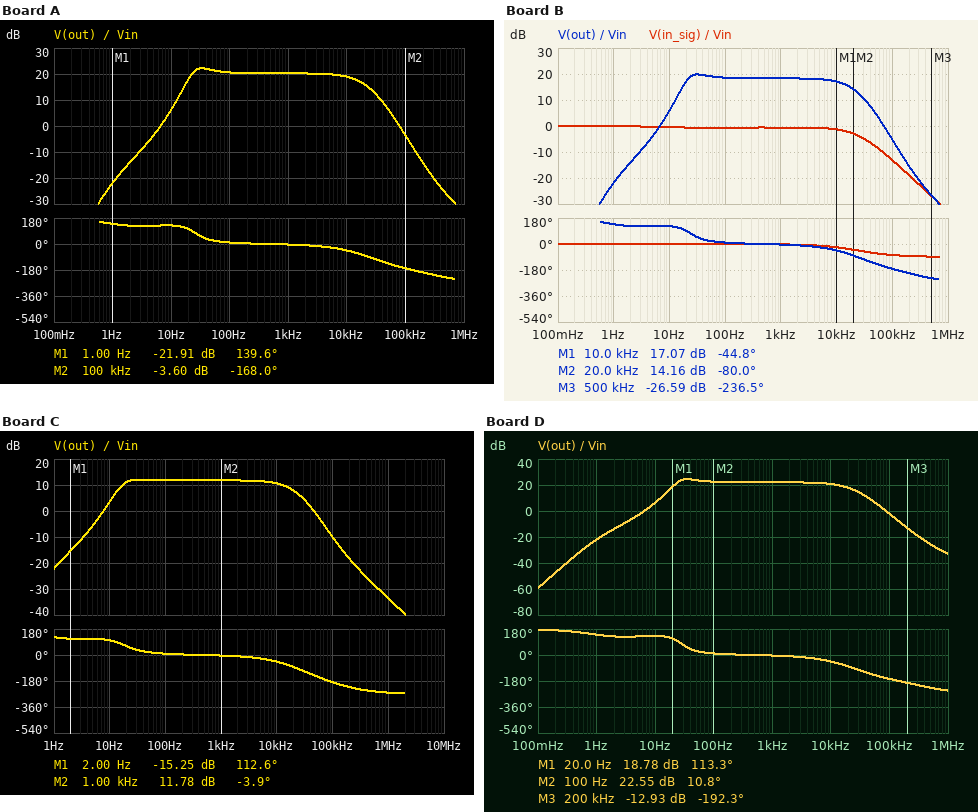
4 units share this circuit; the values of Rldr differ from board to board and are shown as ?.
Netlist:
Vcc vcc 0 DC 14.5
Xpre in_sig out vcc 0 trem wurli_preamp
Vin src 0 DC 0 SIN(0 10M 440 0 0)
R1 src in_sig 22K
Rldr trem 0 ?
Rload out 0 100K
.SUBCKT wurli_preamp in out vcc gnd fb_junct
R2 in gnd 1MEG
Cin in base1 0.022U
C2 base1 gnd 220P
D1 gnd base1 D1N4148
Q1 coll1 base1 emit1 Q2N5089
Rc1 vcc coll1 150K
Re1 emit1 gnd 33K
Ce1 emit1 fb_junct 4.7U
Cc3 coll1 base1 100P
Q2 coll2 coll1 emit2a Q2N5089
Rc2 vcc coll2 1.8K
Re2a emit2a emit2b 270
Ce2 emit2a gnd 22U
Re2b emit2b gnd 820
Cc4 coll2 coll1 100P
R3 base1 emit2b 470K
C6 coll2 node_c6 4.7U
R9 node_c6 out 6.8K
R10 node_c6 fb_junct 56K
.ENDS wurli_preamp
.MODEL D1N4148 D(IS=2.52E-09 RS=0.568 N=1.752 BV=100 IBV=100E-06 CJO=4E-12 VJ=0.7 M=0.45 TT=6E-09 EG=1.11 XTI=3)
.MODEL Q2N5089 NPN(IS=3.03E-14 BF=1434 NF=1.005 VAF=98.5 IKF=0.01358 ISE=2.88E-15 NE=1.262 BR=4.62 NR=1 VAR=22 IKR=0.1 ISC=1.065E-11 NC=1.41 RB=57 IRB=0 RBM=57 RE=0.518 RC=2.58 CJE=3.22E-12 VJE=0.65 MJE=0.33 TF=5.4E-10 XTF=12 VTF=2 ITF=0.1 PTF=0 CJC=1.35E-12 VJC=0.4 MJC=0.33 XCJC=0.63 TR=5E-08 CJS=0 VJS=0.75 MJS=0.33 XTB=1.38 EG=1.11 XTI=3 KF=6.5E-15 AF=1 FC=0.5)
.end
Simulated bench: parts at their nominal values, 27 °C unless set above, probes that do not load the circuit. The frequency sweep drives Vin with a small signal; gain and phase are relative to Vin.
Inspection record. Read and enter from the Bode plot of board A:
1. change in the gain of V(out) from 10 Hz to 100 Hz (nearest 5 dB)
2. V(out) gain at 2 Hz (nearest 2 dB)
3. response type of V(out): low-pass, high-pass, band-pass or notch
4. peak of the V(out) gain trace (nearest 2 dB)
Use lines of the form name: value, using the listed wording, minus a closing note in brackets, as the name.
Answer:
change in the gain of V(out) from 10 Hz to 100 Hz: 15 dB
V(out) gain at 2 Hz: -14 dB
response type of V(out): low-pass, high-pass, band-pass or notch: band-pass
peak of the V(out) gain trace: 22 dB
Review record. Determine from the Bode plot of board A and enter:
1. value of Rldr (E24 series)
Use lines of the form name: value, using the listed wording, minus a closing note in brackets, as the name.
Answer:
value of Rldr: 5.6 kΩ
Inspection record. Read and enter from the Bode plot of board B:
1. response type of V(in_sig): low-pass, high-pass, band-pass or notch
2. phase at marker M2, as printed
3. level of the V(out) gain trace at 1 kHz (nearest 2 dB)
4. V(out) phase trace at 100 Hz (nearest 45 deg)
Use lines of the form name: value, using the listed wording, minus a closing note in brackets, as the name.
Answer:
response type of V(in_sig): low-pass, high-pass, band-pass or notch: low-pass
phase at marker M2, as printed: -80.0 deg
level of the V(out) gain trace at 1 kHz: 18 dB
V(out) phase trace at 100 Hz: 0 deg
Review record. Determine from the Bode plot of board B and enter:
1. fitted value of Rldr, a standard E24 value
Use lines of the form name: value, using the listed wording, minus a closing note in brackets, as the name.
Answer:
fitted value of Rldr, a standard E24 value: 7.5 kΩ
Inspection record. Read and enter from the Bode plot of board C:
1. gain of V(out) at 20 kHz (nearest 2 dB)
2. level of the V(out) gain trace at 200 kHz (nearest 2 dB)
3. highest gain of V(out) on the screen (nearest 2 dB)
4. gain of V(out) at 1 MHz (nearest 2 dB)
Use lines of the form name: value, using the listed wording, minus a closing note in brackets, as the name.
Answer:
gain of V(out) at 20 kHz: 8 dB
level of the V(out) gain trace at 200 kHz: -18 dB
highest gain of V(out) on the screen: 12 dB
gain of V(out) at 1 MHz: -34 dB
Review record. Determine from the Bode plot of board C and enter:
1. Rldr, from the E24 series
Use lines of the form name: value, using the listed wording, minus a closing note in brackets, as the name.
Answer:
Rldr, from the E24 series: 27 kΩ
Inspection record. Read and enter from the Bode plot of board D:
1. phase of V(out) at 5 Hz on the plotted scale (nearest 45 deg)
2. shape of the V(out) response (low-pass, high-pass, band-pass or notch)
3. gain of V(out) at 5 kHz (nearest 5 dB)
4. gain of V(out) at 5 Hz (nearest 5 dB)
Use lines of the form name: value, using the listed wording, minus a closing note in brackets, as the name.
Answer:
phase of V(out) at 5 Hz on the plotted scale: 135 deg
shape of the V(out) response: band-pass
gain of V(out) at 5 kHz: 20 dB
gain of V(out) at 5 Hz: -5 dB
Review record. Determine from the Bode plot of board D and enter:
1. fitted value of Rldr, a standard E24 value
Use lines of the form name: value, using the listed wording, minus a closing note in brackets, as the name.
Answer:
fitted value of Rldr, a standard E24 value: 4.3 kΩ
